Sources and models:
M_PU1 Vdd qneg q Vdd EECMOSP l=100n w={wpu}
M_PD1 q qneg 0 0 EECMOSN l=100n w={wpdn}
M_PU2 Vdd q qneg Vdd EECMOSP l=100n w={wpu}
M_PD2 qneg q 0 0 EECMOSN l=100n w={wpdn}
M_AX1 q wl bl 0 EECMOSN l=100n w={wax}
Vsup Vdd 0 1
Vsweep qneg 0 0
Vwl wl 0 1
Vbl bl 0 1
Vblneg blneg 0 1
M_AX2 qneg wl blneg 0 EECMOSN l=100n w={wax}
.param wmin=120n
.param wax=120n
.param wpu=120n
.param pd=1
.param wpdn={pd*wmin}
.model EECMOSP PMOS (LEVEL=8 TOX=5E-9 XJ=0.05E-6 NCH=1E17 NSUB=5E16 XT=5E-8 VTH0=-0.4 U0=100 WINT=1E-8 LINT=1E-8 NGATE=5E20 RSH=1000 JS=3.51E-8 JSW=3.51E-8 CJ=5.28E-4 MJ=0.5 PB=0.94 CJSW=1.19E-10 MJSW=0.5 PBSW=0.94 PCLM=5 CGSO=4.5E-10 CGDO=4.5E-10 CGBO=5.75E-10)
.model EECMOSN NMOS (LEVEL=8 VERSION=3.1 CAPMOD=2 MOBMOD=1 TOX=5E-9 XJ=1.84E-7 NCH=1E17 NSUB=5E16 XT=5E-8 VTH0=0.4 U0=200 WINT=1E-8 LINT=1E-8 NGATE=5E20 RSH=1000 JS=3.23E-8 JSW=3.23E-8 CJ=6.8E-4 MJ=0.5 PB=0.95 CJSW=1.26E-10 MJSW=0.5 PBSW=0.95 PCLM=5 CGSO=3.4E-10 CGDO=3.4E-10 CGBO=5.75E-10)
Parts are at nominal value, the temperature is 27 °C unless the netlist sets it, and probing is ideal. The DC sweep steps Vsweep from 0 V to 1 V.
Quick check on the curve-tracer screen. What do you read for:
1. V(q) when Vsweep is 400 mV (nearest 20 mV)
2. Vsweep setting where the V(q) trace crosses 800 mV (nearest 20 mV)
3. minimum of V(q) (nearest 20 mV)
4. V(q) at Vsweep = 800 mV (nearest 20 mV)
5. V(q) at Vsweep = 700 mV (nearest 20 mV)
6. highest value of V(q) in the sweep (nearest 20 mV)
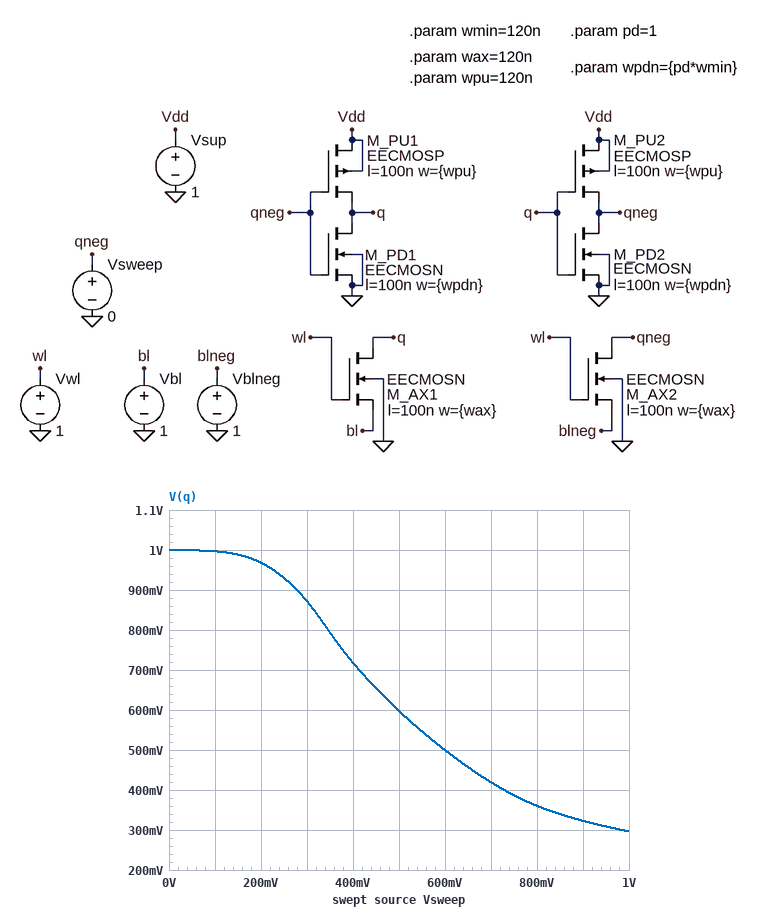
720 mV
340 mV
300 mV
360 mV
420 mV
1.00 V
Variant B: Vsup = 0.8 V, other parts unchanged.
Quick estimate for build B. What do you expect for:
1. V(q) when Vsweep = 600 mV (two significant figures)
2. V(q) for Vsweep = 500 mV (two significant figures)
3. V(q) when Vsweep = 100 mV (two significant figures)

460 mV
530 mV
800 mV
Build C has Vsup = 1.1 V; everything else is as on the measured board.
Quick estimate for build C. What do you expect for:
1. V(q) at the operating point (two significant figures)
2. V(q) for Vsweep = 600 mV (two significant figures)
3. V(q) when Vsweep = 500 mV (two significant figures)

1.1 V
540 mV
650 mV
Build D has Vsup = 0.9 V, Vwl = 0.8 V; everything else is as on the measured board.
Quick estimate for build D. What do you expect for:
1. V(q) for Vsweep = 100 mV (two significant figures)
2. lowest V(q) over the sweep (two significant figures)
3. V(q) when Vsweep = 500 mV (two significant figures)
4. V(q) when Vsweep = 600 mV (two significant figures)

900 mV
210 mV
430 mV
350 mV
